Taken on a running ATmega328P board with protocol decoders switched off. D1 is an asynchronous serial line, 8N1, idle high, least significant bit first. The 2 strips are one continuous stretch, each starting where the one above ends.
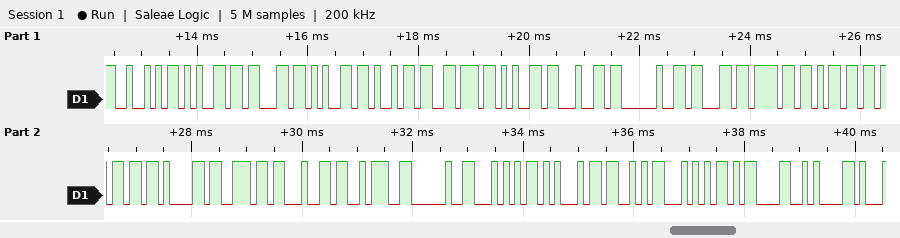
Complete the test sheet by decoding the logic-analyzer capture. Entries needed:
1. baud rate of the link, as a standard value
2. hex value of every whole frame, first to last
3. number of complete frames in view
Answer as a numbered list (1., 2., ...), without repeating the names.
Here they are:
1. 9600 baud
2. 52 65 63 65 69 76 65 64 20 63 6F 6D 6D 61 6E 64 3A 20 54 45 53 54 0D 0A
3. 24
